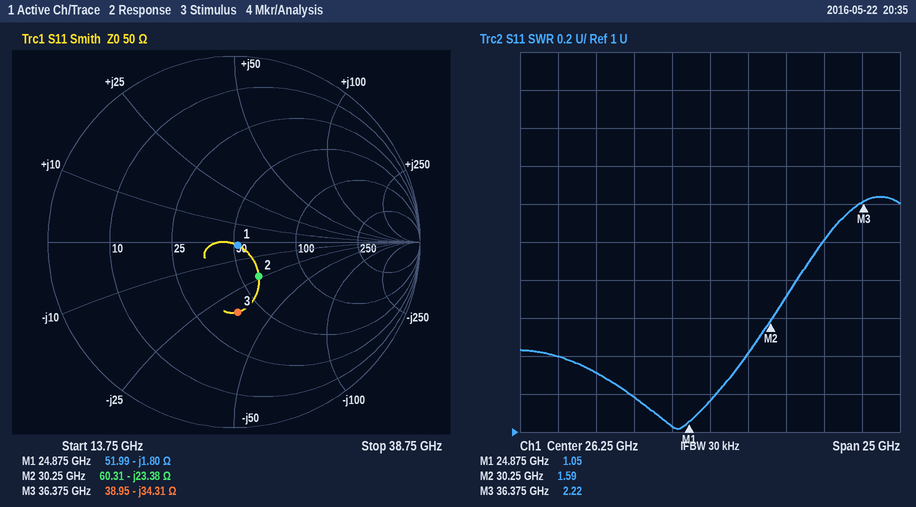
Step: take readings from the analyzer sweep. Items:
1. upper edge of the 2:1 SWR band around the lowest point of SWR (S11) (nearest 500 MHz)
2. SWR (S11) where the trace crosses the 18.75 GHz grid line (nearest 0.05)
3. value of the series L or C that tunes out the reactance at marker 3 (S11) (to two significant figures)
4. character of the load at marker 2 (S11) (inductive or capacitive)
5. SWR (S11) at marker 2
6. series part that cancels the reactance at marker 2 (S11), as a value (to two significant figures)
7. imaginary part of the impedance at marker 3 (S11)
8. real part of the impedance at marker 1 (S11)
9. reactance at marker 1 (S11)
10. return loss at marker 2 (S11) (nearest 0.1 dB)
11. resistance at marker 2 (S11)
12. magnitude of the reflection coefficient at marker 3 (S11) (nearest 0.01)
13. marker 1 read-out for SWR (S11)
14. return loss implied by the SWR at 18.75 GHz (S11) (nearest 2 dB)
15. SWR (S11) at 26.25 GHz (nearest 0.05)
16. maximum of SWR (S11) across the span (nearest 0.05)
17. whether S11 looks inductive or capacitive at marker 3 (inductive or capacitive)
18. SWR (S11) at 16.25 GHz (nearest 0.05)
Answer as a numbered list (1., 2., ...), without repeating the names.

1. 33.5 GHz
2. 1.30
3. 150 pH
4. capacitive
5. 1.59
6. 120 pH
7. -34.31 Ω
8. 51.99 Ω
9. -1.80 Ω
10. 12.9 dB
11. 60.31 Ω
12. 0.38
13. 1.05
14. 18 dB
15. 1.15
16. 2.25
17. capacitive
18. 1.40
